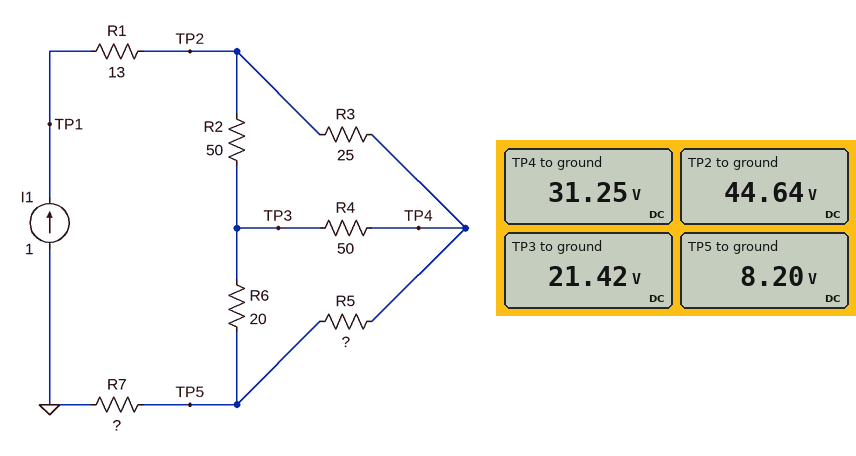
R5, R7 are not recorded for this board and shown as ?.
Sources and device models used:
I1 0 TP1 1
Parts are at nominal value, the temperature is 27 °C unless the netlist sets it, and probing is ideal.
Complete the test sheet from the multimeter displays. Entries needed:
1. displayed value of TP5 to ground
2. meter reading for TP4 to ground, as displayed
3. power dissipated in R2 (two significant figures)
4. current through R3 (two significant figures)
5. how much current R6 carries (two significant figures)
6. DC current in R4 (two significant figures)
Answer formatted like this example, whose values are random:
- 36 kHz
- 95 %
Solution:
- 8.20 V
- 31.25 V
- 11 W
- 540 mA
- 660 mA
- 200 mA
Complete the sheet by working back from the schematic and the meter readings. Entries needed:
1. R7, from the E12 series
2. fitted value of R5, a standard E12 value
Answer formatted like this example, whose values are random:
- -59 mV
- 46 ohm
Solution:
- 8.2 Ω
- 68 Ω
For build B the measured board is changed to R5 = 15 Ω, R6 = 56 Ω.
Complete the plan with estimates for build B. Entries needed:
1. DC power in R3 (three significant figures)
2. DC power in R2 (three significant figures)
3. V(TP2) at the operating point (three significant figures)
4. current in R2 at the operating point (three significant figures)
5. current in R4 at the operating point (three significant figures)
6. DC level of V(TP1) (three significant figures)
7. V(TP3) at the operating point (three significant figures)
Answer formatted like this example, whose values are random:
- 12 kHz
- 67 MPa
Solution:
- 12.3 W
- 4.47 W
- 37.0 V
- 299 mA
- 51.5 mA
- 50.0 V
- 22.1 V
